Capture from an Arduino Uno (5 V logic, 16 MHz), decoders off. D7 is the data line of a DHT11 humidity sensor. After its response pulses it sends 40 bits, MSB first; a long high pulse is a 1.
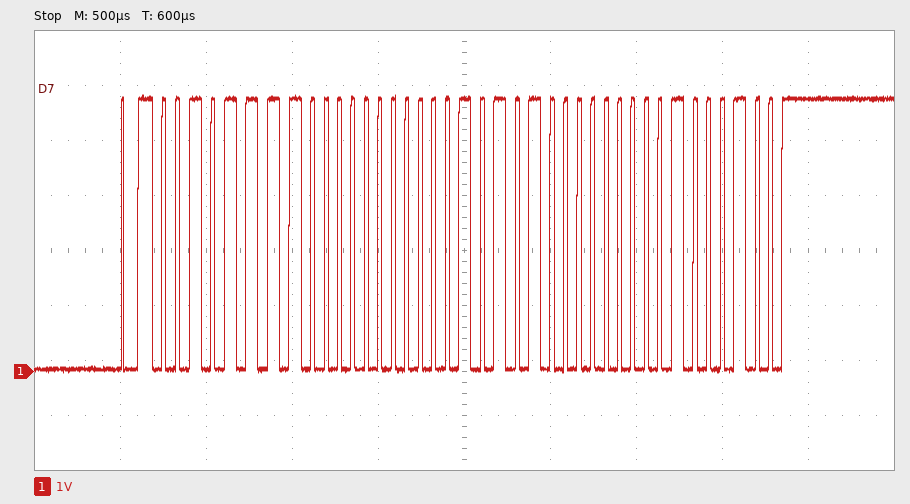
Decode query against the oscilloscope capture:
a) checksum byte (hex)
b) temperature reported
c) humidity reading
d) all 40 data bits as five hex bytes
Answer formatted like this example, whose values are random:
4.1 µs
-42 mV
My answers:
0x44
21.0 °C
47 %
2F 00 15 00 44
